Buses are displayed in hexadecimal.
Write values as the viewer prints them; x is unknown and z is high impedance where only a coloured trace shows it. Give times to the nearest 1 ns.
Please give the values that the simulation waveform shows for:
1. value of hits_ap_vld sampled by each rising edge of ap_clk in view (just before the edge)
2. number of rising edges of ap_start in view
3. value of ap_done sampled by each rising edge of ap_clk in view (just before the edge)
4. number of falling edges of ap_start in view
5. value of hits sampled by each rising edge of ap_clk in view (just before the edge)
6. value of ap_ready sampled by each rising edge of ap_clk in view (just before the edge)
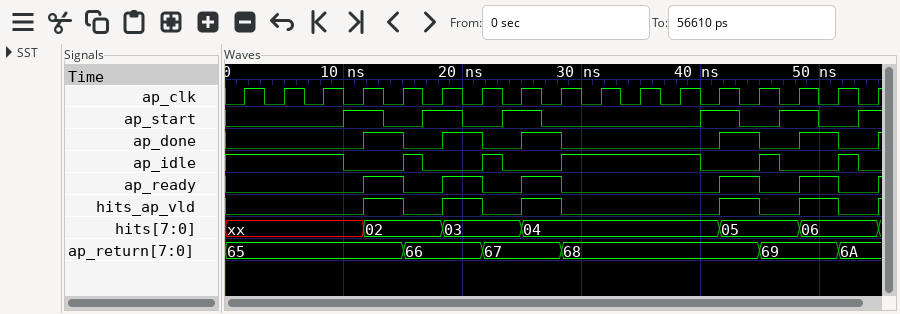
0 0 0 0 1 0 1 0 1 0 0 0 0 1 0 1 0
6
0 0 0 0 1 0 1 0 1 0 0 0 0 1 0 1 0
5
xx, xx, xx, xx, 02, 02, 03, 03, 04, 04, 04, 04, 04, 05, 05, 06, 06
0 0 0 0 1 0 1 0 1 0 0 0 0 1 0 1 0
